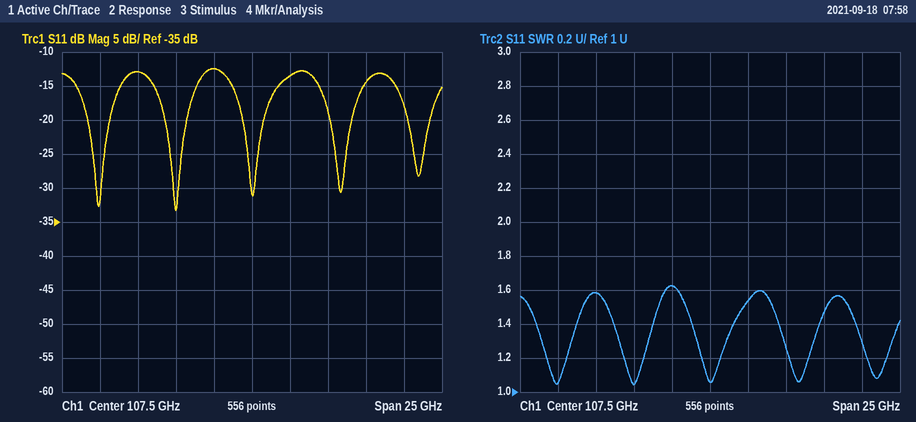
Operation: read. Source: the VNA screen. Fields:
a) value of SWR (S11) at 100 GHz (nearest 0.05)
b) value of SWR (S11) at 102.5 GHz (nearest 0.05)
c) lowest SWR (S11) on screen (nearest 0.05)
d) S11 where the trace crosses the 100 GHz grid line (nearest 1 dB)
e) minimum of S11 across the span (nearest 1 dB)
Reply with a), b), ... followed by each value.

a) 1.60
b) 1.05
c) 1.05
d) -13 dB
e) -33 dB
